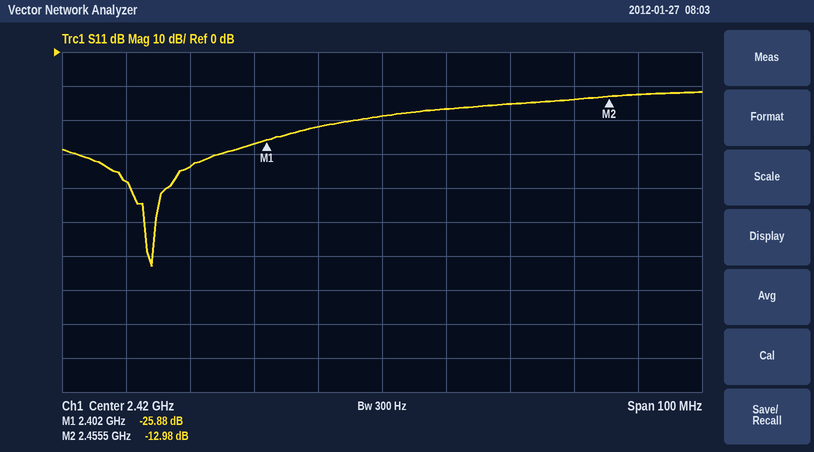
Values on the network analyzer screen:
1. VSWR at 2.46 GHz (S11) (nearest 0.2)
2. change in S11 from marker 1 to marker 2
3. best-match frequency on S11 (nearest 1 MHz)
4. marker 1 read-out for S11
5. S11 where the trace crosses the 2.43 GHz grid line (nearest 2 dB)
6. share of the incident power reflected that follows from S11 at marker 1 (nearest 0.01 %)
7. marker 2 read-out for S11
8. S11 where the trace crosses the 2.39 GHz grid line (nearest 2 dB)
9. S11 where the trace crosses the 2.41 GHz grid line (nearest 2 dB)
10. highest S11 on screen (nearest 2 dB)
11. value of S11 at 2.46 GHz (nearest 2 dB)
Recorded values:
1.6
12.90 dB
2.384 GHz
-25.88 dB
-16 dB
0.26 %
-12.98 dB
-34 dB
-22 dB
-12 dB
-12 dB
